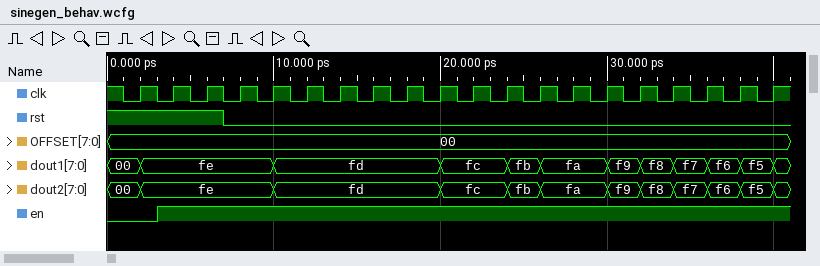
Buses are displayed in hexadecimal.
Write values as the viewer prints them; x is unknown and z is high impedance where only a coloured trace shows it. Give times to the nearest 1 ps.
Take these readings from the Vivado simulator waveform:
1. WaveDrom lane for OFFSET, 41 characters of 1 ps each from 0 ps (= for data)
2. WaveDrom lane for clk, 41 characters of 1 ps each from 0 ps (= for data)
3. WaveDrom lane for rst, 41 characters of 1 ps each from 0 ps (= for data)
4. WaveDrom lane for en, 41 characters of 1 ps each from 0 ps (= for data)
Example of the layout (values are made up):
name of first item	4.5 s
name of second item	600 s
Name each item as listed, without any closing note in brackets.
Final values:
WaveDrom lane for OFFSET, 41 characters of 1 ps each from 0 ps	{name: 'OFFSET', wave: '=........................................', data: '00'}
WaveDrom lane for clk, 41 characters of 1 ps each from 0 ps	{name: 'clk', wave: '10101010101010101010101010101010101010101'}
WaveDrom lane for rst, 41 characters of 1 ps each from 0 ps	{name: 'rst', wave: '1......0.................................'}
WaveDrom lane for en, 41 characters of 1 ps each from 0 ps	{name: 'en', wave: '0..1.....................................'}
